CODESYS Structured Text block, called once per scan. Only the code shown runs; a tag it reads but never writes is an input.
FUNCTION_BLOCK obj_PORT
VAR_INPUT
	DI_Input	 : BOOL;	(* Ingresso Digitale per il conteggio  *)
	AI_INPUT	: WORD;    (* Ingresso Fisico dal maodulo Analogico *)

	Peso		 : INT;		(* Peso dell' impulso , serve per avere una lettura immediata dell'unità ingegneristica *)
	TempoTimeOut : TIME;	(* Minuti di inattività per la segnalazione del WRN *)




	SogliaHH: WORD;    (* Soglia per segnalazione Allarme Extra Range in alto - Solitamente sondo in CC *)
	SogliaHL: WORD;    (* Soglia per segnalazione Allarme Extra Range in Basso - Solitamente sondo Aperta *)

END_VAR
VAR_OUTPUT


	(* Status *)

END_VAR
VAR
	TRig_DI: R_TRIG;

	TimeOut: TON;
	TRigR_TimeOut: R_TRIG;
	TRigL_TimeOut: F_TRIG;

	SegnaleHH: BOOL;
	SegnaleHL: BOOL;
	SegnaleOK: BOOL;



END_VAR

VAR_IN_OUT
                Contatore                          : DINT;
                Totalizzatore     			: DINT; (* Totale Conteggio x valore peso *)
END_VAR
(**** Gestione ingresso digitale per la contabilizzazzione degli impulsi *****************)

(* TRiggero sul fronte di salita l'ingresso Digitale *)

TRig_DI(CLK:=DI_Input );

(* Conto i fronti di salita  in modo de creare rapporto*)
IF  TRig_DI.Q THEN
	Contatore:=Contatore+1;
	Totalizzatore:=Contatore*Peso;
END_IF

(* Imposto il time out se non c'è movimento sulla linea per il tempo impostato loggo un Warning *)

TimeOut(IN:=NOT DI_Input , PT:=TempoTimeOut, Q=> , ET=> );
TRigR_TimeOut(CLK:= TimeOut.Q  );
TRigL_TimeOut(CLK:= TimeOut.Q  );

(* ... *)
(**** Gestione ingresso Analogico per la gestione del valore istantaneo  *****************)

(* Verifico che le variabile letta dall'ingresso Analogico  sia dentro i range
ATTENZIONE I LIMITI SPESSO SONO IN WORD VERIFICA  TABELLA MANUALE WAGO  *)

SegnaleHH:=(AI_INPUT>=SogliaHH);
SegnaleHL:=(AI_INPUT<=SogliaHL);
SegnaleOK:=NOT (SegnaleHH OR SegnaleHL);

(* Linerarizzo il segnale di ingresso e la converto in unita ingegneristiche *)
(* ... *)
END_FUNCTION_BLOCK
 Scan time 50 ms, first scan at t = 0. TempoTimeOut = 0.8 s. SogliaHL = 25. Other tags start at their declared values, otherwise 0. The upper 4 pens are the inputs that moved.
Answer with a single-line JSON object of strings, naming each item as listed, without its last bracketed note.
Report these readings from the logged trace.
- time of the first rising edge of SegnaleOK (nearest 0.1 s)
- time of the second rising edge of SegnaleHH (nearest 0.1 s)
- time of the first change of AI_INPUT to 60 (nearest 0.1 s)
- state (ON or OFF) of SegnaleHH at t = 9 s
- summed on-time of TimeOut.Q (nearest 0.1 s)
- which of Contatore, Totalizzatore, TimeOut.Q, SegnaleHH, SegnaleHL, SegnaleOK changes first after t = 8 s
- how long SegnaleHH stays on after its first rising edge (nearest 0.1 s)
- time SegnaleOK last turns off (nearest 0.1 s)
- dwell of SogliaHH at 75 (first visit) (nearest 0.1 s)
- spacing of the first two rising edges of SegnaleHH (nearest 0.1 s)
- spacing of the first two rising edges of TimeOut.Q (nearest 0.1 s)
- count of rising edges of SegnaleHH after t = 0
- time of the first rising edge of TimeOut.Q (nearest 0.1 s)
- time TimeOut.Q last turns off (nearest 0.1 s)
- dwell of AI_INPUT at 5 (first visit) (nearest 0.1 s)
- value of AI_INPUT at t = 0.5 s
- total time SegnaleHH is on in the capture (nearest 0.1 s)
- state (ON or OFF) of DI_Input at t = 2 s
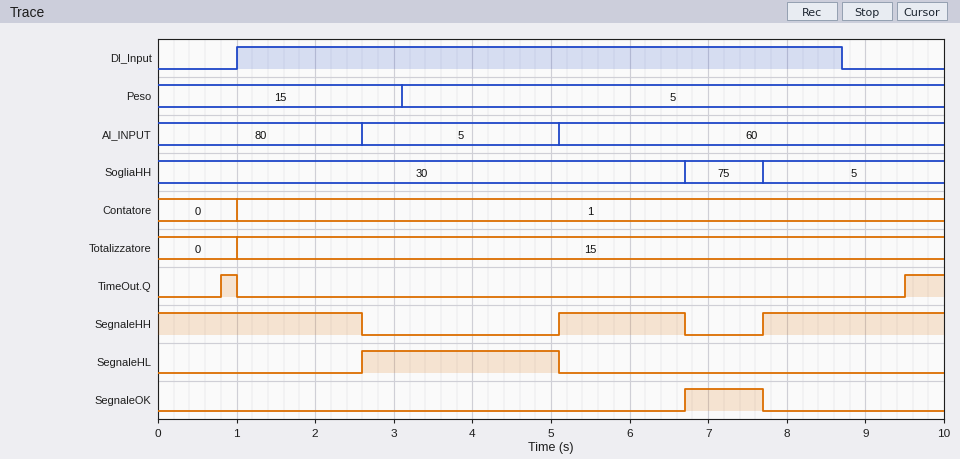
{"time of the first rising edge of SegnaleOK": "6.7 s", "time of the second rising edge of SegnaleHH": "7.7 s", "time of the first change of AI_INPUT to 60": "5.1 s", "state (ON or OFF) of SegnaleHH at t = 9 s": "ON", "summed on-time of TimeOut.Q": "0.7 s", "which of Contatore, Totalizzatore, TimeOut.Q, SegnaleHH, SegnaleHL, SegnaleOK changes first after t = 8 s": "TimeOut.Q", "how long SegnaleHH stays on after its first rising edge": "1.6 s", "time SegnaleOK last turns off": "7.7 s", "dwell of SogliaHH at 75 (first visit)": "1.0 s", "spacing of the first two rising edges of SegnaleHH": "2.6 s", "spacing of the first two rising edges of TimeOut.Q": "8.7 s", "count of rising edges of SegnaleHH after t = 0": "2", "time of the first rising edge of TimeOut.Q": "0.8 s", "time TimeOut.Q last turns off": "1.0 s", "dwell of AI_INPUT at 5 (first visit)": "2.5 s", "value of AI_INPUT at t = 0.5 s": "80", "total time SegnaleHH is on in the capture": "6.5 s", "state (ON or OFF) of DI_Input at t = 2 s": "ON"}
